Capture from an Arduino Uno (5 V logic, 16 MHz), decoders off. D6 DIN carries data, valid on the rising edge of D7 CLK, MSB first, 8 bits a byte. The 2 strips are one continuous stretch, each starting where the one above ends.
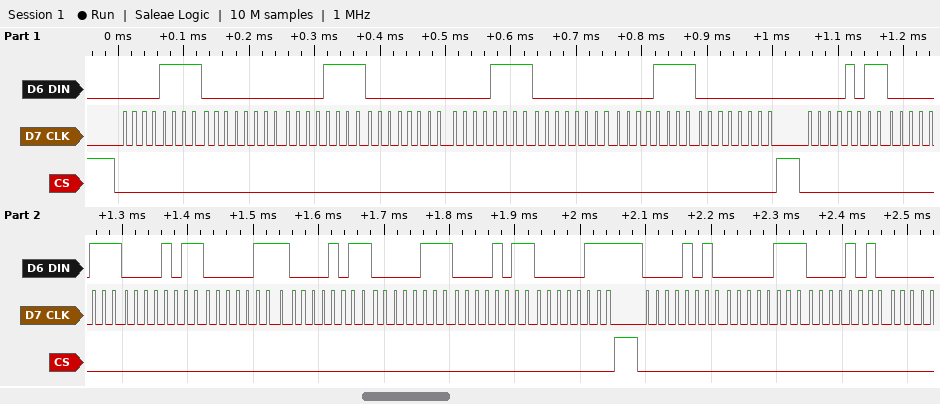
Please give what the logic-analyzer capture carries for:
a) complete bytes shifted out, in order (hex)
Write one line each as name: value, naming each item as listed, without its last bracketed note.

complete bytes shifted out, in order: 0F 00 0F 00 0F 00 0F 00 0B 07 0B 07 0B 07 0B 07 0A 07 0A
